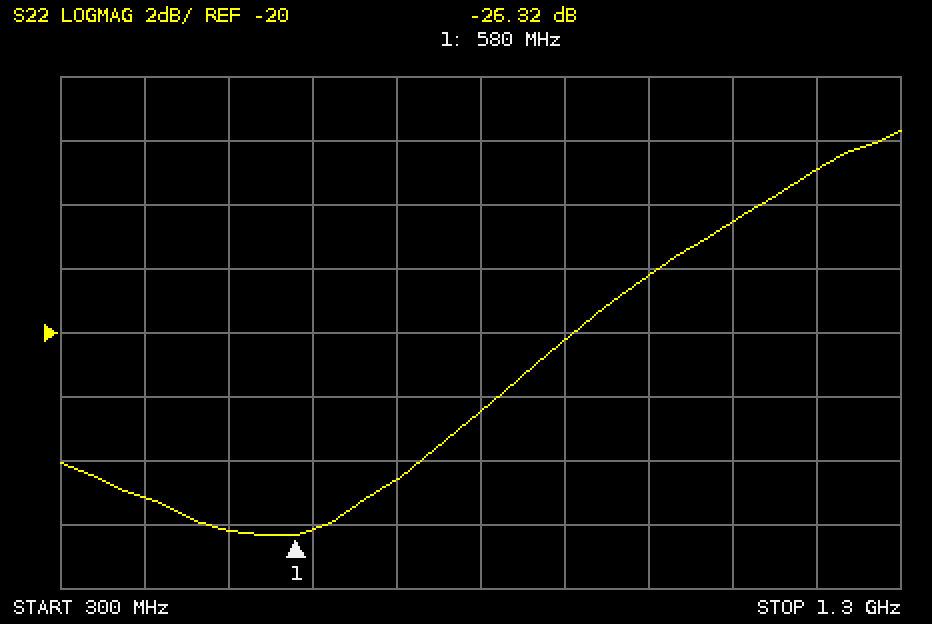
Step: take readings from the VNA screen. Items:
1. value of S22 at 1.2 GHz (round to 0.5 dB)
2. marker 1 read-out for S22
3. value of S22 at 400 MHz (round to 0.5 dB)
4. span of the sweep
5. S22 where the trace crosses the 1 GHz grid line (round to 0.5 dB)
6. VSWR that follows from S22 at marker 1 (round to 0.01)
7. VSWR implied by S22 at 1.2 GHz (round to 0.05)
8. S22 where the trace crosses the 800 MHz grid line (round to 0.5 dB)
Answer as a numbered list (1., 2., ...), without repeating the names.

1. -15.0 dB
2. -26.32 dB
3. -25.0 dB
4. 1 GHz
5. -18.0 dB
6. 1.10
7. 1.45
8. -22.5 dB
